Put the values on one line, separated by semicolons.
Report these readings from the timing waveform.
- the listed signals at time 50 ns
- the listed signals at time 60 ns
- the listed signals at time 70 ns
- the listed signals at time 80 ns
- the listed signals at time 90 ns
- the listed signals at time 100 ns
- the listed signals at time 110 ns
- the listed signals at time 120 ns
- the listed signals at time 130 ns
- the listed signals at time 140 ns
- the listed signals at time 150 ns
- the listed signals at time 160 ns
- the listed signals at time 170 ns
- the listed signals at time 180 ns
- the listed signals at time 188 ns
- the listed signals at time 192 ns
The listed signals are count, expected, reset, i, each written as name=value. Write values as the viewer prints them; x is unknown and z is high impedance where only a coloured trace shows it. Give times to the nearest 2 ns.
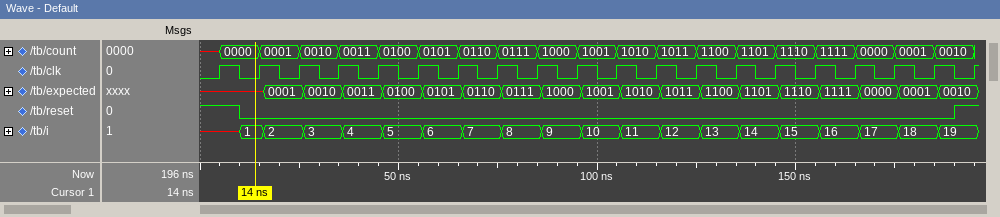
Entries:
count=0100, expected=0100, reset=0, i=5; count=0101, expected=0101, reset=0, i=6; count=0110, expected=0110, reset=0, i=7; count=0111, expected=0111, reset=0, i=8; count=1000, expected=1000, reset=0, i=9; count=1001, expected=1001, reset=0, i=10; count=1010, expected=1010, reset=0, i=11; count=1011, expected=1011, reset=0, i=12; count=1100, expected=1100, reset=0, i=13; count=1101, expected=1101, reset=0, i=14; count=1110, expected=1110, reset=0, i=15; count=1111, expected=1111, reset=0, i=16; count=0000, expected=0000, reset=0, i=17; count=0001, expected=0001, reset=0, i=18; count=0010, expected=0010, reset=0, i=19; count=0010, expected=0010, reset=1, i=19
